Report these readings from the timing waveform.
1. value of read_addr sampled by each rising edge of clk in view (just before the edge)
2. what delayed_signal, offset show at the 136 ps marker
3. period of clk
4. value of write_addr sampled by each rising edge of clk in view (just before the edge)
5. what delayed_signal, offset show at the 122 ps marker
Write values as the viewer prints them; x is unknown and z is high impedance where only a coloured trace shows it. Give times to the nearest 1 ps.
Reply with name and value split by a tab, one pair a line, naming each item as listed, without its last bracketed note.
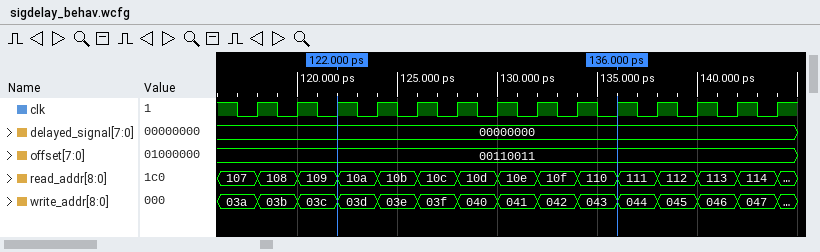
value of read_addr sampled by each rising edge of clk in view	107, 108, 109, 10a, 10b, 10c, 10d, 10e, 10f, 110, 111, 112, 113, 114
what delayed_signal, offset show at the 136 ps marker	delayed_signal=00000000, offset=00110011
period of clk	2 ps
value of write_addr sampled by each rising edge of clk in view	03a, 03b, 03c, 03d, 03e, 03f, 040, 041, 042, 043, 044, 045, 046, 047
what delayed_signal, offset show at the 122 ps marker	delayed_signal=00000000, offset=00110011
